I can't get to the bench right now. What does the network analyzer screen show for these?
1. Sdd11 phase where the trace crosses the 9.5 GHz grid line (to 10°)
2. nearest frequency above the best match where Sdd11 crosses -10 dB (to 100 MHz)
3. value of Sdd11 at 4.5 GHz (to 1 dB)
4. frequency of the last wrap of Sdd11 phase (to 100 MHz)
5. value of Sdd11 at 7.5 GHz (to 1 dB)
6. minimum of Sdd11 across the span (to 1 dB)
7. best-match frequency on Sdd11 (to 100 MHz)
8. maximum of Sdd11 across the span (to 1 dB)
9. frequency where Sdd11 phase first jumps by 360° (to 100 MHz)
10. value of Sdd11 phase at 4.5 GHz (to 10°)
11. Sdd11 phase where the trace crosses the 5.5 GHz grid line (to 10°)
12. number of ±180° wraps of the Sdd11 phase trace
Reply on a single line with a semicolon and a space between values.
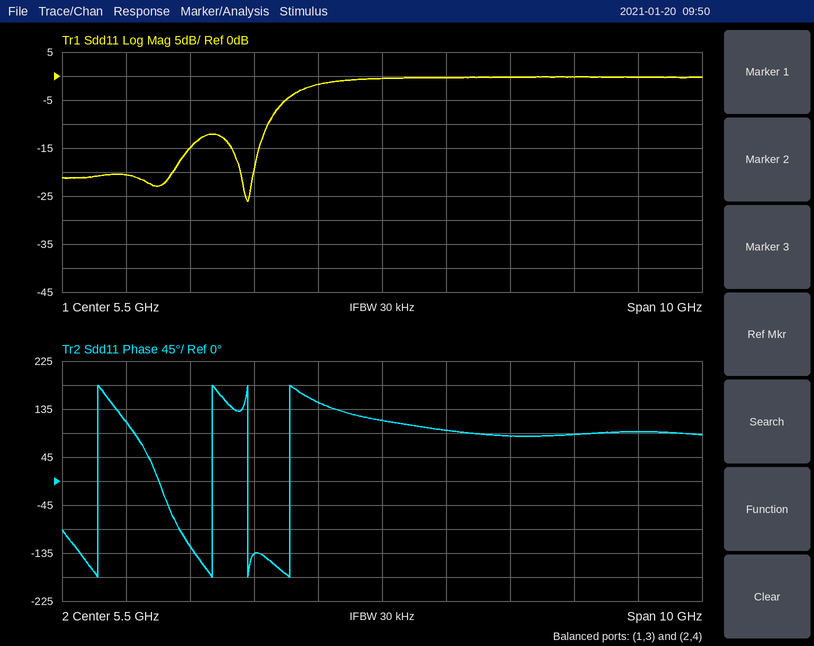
90°; 3.7 GHz; -2 dB; 4.1 GHz; 0 dB; -26 dB; 3.4 GHz; 0 dB; 1.1 GHz; 150°; 110°; 4
